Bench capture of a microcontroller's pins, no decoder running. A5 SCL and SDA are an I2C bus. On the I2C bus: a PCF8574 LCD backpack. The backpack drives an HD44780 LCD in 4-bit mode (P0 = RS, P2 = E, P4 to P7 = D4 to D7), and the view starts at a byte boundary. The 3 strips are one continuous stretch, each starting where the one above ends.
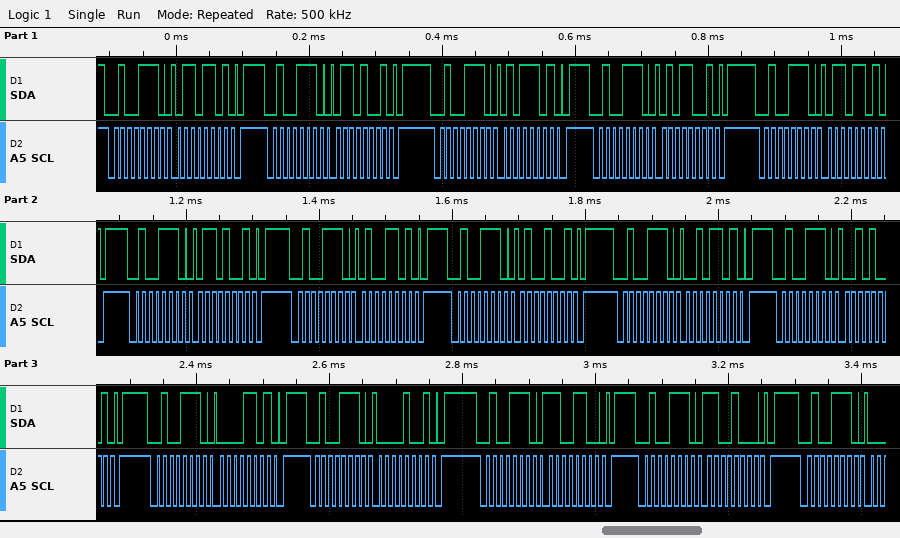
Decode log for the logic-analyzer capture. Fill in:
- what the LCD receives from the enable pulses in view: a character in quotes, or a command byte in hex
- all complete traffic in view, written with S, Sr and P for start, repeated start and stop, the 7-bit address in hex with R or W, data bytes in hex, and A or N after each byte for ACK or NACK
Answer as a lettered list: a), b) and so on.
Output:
a) 'e' 'd' ' '
b) S 27W A 6D A P S 27W A 69 A P S 27W A 5D A P S 27W A 59 A P S 27W A 6D A P S 27W A 69 A P S 27W A 4D A P S 27W A 49 A P S 27W A 2D A P S 27W A 29 A P S 27W A 0D A P S 27W A 09 A P S 27W A CC A P S 27W A C8 A P S 27W A
